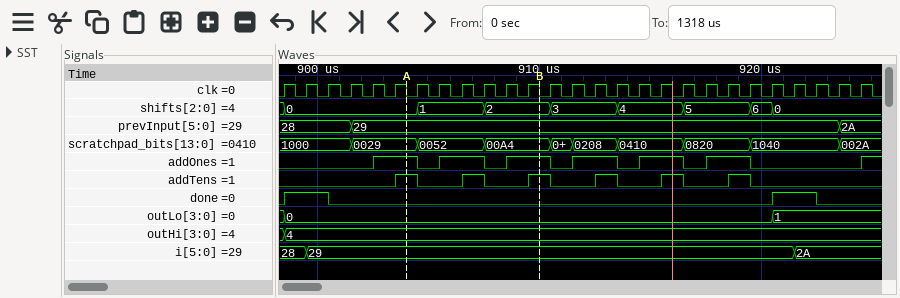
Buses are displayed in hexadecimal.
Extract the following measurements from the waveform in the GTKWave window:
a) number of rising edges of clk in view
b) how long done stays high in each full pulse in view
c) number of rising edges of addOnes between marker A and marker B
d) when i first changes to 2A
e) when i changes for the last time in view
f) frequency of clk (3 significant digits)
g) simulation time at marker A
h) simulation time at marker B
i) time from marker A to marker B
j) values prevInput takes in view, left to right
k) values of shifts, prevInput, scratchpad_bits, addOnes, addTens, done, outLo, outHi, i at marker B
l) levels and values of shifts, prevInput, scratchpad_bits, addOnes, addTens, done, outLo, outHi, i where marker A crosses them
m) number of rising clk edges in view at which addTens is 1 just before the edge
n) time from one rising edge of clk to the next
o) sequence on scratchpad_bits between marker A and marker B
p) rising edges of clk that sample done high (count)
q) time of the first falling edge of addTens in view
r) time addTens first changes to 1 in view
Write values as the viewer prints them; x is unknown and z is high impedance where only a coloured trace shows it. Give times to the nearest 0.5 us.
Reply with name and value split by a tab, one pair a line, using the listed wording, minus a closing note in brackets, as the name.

number of rising edges of clk in view	27
how long done stays high in each full pulse in view	2 us, 2 us
number of rising edges of addOnes between marker A and marker B	2
when i first changes to 2A	921.5 us
when i changes for the last time in view	921.5 us
frequency of clk	1.00 MHz
simulation time at marker A	904 us
simulation time at marker B	910 us
time from marker A to marker B	6 us
values prevInput takes in view, left to right	28, 29, 2A
values of shifts, prevInput, scratchpad_bits, addOnes, addTens, done, outLo, outHi, i at marker B	shifts=2, prevInput=29, scratchpad_bits=00A4, addOnes=1, addTens=1, done=0, outLo=0, outHi=4, i=29
levels and values of shifts, prevInput, scratchpad_bits, addOnes, addTens, done, outLo, outHi, i where marker A crosses them	shifts=0, prevInput=29, scratchpad_bits=0029, addOnes=1, addTens=1, done=0, outLo=0, outHi=4, i=29
number of rising clk edges in view at which addTens is 1 just before the edge	6
time from one rising edge of clk to the next	1 us
sequence on scratchpad_bits between marker A and marker B	0029, 0052, 00A4
rising edges of clk that sample done high	4
time of the first falling edge of addTens in view	904.5 us
time addTens first changes to 1 in view	903.5 us
